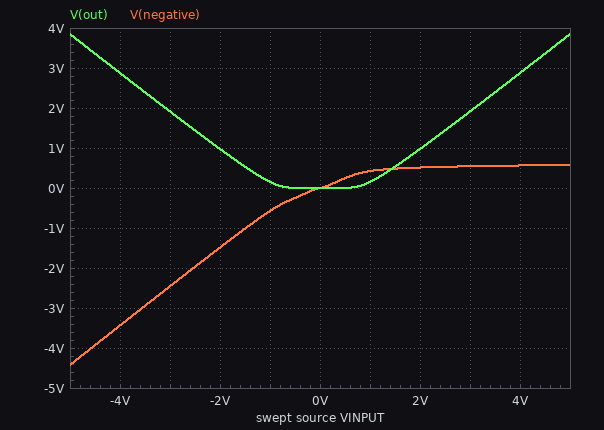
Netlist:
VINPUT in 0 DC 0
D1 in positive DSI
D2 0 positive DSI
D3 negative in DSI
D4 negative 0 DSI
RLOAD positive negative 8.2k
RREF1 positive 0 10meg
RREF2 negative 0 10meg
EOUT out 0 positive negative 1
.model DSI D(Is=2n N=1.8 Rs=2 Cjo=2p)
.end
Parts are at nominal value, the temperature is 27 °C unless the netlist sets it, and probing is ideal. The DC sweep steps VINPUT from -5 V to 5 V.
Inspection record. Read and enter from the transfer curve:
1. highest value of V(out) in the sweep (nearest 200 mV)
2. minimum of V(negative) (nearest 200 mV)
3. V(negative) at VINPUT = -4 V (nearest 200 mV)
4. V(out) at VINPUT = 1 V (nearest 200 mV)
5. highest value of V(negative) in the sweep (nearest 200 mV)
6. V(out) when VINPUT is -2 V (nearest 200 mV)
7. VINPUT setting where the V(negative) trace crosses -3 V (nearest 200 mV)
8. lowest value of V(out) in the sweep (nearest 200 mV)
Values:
3.8 V
-4.4 V
-3.4 V
200 mV
600 mV
1.0 V
-3.6 V
0 V
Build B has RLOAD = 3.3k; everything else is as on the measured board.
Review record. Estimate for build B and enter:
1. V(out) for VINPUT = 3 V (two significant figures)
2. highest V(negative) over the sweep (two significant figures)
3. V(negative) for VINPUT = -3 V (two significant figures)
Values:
1.8 V
620 mV
-2.4 V
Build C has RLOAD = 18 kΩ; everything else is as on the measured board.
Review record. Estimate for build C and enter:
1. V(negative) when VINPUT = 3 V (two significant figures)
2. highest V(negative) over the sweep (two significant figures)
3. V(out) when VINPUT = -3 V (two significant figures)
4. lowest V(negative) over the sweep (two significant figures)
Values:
510 mV
540 mV
2.0 V
-4.5 V
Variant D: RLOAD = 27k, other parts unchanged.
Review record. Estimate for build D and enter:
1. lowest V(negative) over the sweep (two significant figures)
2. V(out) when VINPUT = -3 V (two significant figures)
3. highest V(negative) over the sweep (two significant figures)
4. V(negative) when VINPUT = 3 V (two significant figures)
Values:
-4.5 V
2.0 V
520 mV
490 mV
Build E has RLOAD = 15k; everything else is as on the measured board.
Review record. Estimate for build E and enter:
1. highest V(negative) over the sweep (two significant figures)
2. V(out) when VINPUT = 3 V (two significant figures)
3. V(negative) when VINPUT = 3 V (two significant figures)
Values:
550 mV
2.0 V
520 mV
